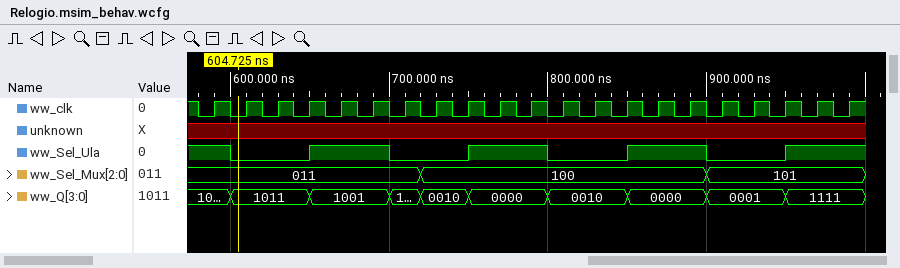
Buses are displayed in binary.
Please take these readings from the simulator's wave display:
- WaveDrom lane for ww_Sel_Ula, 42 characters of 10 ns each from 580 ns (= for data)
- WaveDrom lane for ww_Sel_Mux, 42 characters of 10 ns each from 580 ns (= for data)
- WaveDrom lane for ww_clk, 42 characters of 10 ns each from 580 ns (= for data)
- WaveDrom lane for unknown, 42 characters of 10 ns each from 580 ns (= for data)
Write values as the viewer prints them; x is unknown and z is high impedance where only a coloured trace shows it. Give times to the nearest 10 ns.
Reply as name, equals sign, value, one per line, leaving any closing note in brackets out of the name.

WaveDrom lane for ww_Sel_Ula, 42 characters of 10 ns each from 580 ns = {name: 'ww_Sel_Ula', wave: '1.0....1....0....1....0....1....0....1....'}
WaveDrom lane for ww_Sel_Mux, 42 characters of 10 ns each from 580 ns = {name: 'ww_Sel_Mux', wave: '=.............=.................=.........', data: '011 100 101'}
WaveDrom lane for ww_clk, 42 characters of 10 ns each from 580 ns = {name: 'ww_clk', wave: '010101010101010101010101010101010101010101'}
WaveDrom lane for unknown, 42 characters of 10 ns each from 580 ns = {name: 'unknown', wave: 'x.........................................'}
